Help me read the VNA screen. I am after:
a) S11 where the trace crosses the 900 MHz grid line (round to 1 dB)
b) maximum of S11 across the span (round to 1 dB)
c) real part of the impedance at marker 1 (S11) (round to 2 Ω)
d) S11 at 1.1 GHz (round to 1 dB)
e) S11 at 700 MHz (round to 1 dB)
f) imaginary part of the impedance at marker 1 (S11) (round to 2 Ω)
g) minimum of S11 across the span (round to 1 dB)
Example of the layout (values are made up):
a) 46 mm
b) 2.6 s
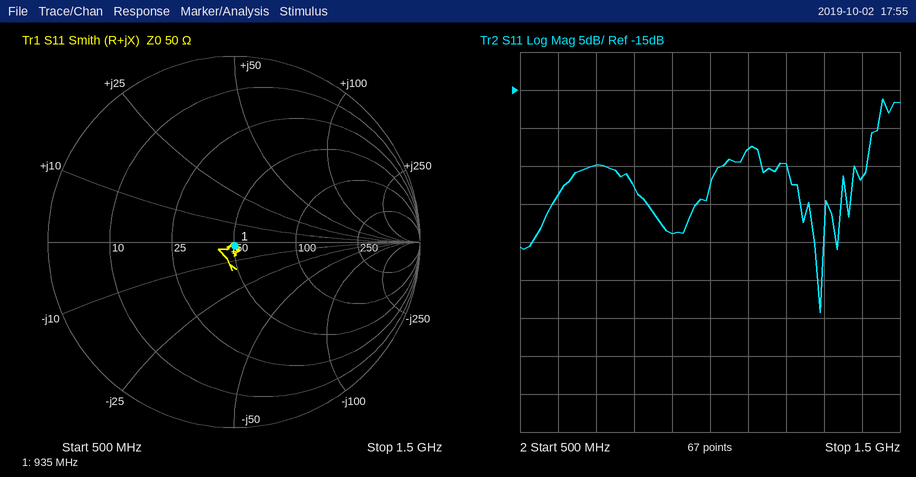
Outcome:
a) -34 dB
b) -16 dB
c) 50 Ω
d) -23 dB
e) -25 dB
f) -2 Ω
g) -44 dB
